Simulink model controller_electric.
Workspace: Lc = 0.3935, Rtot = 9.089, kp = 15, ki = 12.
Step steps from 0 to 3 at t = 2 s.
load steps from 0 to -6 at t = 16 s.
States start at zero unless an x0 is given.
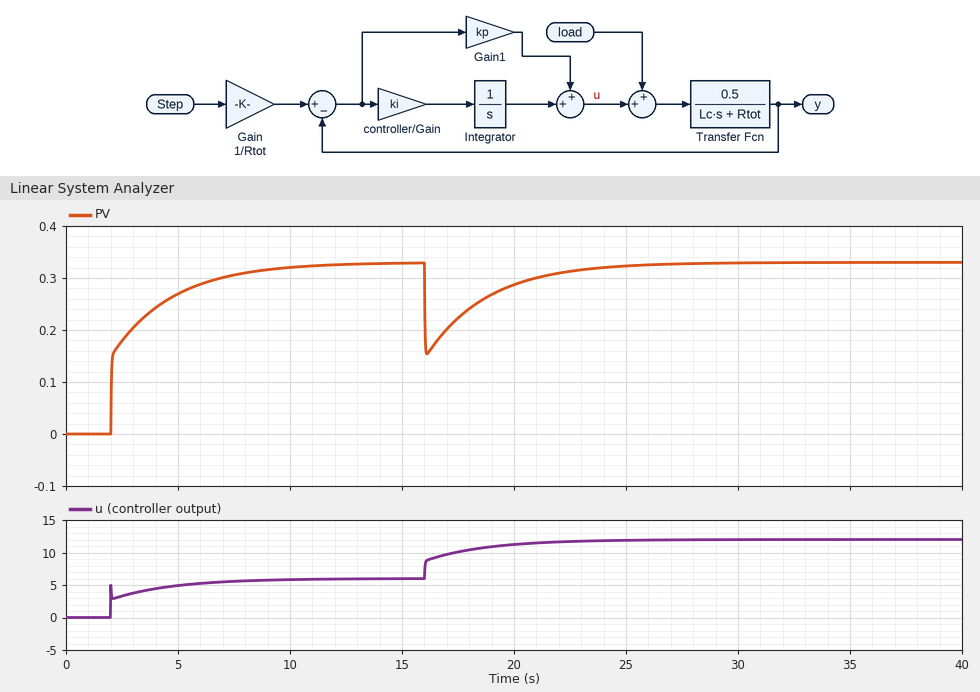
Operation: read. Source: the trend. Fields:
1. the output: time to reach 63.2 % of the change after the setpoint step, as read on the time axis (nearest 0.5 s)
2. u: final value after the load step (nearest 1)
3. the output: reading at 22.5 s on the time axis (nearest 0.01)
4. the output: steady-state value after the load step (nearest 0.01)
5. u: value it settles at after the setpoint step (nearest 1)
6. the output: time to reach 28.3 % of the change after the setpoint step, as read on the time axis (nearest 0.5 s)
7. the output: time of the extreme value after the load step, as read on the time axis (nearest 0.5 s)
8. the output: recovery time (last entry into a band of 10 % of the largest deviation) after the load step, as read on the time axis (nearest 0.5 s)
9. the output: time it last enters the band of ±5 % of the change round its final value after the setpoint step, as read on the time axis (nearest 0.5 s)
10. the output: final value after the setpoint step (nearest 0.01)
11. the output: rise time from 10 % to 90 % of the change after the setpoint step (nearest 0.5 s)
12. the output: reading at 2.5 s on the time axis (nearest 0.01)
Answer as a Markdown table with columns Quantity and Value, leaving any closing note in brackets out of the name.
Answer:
| Quantity | Value |
|---|---|
| the output: time to reach 63.2 % of the change after the setpoint step, as read on the time axis | 3.0 s |
| u: final value after the load step | 12 |
| the output: reading at 22.5 s on the time axis | 0.31 |
| the output: steady-state value after the load step | 0.33 |
| u: value it settles at after the setpoint step | 6 |
| the output: time to reach 28.3 % of the change after the setpoint step, as read on the time axis | 2.0 s |
| the output: time of the extreme value after the load step, as read on the time axis | 16.0 s |
| the output: recovery time (last entry into a band of 10 % of the largest deviation) after the load step, as read on the time axis | 22.5 s |
| the output: time it last enters the band of ±5 % of the change round its final value after the setpoint step, as read on the time axis | 8.5 s |
| the output: final value after the setpoint step | 0.33 |
| the output: rise time from 10 % to 90 % of the change after the setpoint step | 4.5 s |
| the output: reading at 2.5 s on the time axis | 0.18 |
